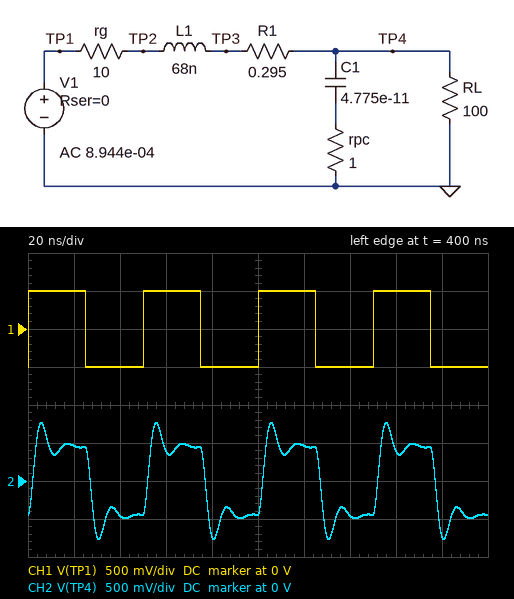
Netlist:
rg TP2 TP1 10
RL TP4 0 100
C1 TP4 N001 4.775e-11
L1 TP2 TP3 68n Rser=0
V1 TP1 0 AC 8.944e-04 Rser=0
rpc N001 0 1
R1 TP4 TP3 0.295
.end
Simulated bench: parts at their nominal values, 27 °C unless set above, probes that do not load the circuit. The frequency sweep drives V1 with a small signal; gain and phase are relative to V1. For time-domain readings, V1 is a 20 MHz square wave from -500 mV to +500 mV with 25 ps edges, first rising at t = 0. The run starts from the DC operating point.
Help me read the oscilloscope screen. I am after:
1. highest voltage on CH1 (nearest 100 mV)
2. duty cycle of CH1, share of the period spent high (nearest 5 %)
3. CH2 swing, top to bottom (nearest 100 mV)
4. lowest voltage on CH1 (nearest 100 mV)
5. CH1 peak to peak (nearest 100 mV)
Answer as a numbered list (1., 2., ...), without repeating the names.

1. 500 mV
2. 50 %
3. 1.5 V
4. -500 mV
5. 1.0 V
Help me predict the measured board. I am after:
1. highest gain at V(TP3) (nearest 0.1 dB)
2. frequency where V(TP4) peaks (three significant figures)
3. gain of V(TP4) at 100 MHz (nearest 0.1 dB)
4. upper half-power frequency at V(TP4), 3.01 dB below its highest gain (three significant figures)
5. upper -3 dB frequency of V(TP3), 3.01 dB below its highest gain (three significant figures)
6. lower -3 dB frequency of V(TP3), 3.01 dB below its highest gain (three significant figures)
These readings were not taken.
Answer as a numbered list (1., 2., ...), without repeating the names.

1. 3.5 dB
2. 82.2 MHz
3. 2.0 dB
4. 109 MHz
5. 109 MHz
6. 39.6 MHz
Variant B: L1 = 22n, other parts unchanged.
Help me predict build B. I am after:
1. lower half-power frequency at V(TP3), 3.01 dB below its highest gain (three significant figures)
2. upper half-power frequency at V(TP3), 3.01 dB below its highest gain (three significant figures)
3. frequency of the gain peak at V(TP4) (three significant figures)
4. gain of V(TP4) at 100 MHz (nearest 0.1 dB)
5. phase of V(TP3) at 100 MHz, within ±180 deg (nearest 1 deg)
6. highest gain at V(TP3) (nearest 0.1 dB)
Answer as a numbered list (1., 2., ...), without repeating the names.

1. 49.0 MHz
2. 193 MHz
3. 141 MHz
4. 1.6 dB
5. -33 deg
6. 2.8 dB
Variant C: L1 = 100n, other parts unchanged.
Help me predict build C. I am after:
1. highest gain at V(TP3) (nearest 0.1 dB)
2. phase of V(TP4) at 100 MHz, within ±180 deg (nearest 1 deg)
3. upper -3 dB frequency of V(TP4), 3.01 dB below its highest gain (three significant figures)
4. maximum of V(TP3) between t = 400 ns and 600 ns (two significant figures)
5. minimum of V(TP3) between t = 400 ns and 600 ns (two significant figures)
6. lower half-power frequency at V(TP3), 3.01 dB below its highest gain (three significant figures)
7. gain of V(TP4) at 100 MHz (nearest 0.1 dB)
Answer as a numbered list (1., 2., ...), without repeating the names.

1. 3.2 dB
2. -128 deg
3. 90.3 MHz
4. 750 mV
5. -750 mV
6. 29.0 MHz
7. -2.0 dB
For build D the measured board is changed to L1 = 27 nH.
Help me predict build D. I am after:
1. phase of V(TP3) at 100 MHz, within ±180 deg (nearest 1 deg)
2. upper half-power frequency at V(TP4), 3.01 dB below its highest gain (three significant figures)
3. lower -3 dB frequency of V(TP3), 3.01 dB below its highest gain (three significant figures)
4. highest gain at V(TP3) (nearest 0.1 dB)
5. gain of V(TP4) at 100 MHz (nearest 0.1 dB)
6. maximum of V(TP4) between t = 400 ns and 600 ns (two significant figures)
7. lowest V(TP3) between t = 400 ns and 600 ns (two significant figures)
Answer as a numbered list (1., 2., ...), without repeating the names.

1. -39 deg
2. 174 MHz
3. 53.1 MHz
4. 3.1 dB
5. 2.2 dB
6. 750 mV
7. -750 mV
